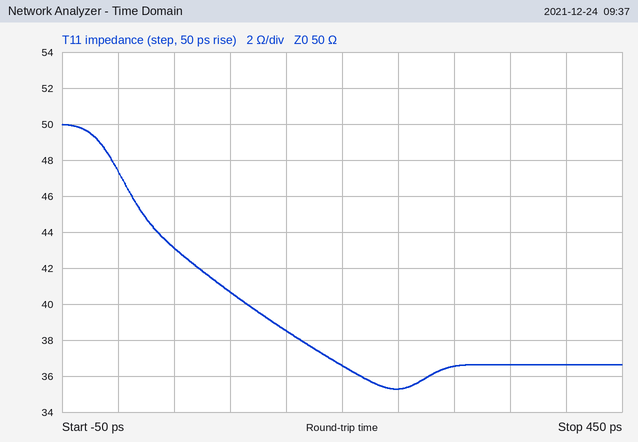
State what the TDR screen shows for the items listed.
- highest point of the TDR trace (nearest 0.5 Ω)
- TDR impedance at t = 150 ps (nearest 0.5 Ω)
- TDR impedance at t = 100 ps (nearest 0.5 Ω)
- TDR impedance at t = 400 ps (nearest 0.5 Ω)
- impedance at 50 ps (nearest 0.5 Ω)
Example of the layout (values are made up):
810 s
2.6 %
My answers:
50.0 Ω
38.5 Ω
40.5 Ω
36.5 Ω
43.0 Ω
